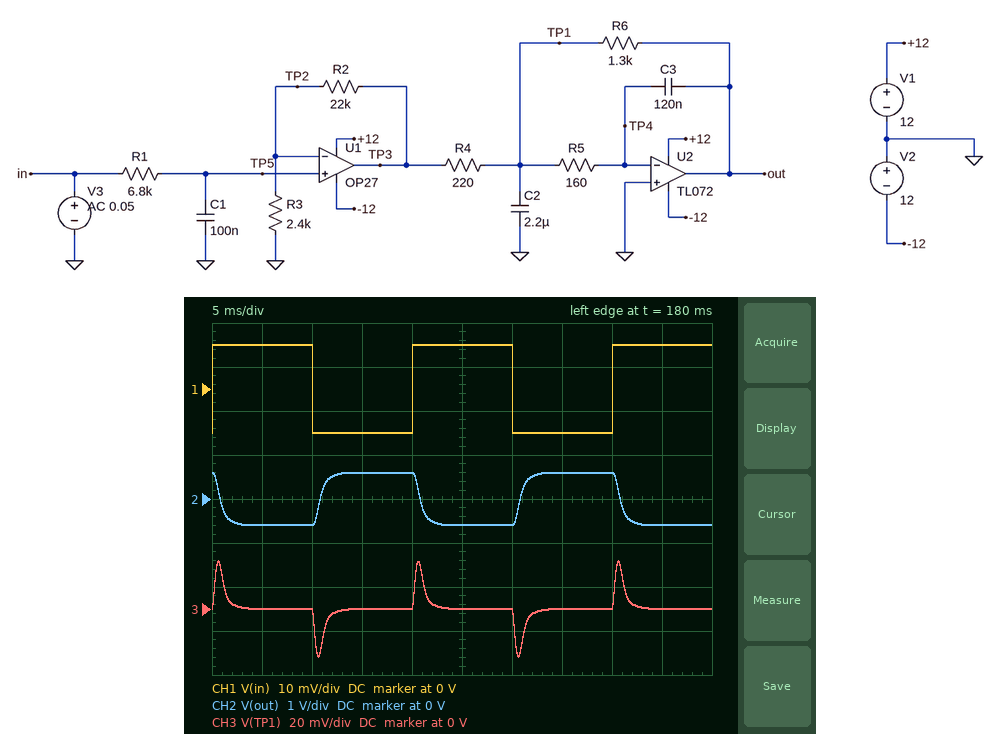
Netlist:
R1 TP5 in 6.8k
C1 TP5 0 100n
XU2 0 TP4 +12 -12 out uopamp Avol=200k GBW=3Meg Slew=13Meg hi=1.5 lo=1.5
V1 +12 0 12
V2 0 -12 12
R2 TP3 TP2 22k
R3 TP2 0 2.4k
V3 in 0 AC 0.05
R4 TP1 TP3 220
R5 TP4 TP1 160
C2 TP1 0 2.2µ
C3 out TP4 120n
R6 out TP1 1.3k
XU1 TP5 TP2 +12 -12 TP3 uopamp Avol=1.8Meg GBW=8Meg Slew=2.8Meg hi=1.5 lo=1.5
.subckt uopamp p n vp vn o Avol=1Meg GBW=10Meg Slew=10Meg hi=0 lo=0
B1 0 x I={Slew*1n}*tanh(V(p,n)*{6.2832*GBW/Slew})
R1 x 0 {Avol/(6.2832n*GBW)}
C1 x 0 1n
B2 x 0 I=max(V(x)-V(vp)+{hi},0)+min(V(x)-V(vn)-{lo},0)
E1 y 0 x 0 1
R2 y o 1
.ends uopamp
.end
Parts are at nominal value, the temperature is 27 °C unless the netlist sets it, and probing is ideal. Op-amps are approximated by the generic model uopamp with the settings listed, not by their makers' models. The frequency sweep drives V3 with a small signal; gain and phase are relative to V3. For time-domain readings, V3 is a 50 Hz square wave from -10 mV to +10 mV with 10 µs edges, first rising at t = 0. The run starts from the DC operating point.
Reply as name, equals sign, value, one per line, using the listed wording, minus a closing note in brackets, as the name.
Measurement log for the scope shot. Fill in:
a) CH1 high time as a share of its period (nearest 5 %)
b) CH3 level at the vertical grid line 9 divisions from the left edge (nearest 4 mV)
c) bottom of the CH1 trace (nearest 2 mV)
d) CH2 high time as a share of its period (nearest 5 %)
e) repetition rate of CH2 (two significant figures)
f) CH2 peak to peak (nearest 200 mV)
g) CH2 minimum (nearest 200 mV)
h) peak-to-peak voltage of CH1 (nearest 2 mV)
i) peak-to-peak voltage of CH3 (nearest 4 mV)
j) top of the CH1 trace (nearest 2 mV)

CH1 high time as a share of its period = 50 %
CH3 level at the vertical grid line 9 divisions from the left edge = 0 V
bottom of the CH1 trace = -10 mV
CH2 high time as a share of its period = 50 %
repetition rate of CH2 = 50 Hz
CH2 peak to peak = 1.2 V
CH2 minimum = -600 mV
peak-to-peak voltage of CH1 = 20 mV
peak-to-peak voltage of CH3 = 44 mV
top of the CH1 trace = 10 mV
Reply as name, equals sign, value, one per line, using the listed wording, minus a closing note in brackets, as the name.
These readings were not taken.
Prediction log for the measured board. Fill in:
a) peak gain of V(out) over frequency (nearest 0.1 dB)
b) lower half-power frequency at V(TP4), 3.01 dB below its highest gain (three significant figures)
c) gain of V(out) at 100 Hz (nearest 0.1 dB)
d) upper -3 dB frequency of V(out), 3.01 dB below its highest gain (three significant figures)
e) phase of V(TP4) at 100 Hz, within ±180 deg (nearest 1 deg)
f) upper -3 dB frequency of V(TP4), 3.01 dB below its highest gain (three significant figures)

peak gain of V(out) over frequency = 35.6 dB
lower half-power frequency at V(TP4), 3.01 dB below its highest gain = 186 Hz
gain of V(out) at 100 Hz = 34.9 dB
upper -3 dB frequency of V(out), 3.01 dB below its highest gain = 245 Hz
phase of V(TP4) at 100 Hz, within ±180 deg = 48 deg
upper -3 dB frequency of V(TP4), 3.01 dB below its highest gain = 804 Hz
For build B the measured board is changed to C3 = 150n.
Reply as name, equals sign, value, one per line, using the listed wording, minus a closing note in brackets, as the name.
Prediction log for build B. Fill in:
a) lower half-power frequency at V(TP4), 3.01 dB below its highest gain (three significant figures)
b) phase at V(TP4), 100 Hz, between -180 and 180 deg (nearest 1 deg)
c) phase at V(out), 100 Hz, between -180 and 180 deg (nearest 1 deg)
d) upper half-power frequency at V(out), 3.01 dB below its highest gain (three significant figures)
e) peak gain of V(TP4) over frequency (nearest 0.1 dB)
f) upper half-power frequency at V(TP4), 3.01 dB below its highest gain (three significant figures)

lower half-power frequency at V(TP4), 3.01 dB below its highest gain = 162 Hz
phase at V(TP4), 100 Hz, between -180 and 180 deg = 45 deg
phase at V(out), 100 Hz, between -180 and 180 deg = 144 deg
upper half-power frequency at V(out), 3.01 dB below its highest gain = 233 Hz
peak gain of V(TP4) over frequency = -48.4 dB
upper half-power frequency at V(TP4), 3.01 dB below its highest gain = 713 Hz
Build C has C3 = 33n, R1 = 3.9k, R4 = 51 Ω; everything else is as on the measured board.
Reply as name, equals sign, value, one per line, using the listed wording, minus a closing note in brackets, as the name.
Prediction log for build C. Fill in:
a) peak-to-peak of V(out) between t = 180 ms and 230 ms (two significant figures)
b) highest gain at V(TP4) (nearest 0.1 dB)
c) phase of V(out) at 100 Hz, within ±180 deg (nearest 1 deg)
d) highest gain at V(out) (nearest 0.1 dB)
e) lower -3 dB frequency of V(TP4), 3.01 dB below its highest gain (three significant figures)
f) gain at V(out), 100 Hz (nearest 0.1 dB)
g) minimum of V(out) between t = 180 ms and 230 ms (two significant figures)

peak-to-peak of V(out) between t = 180 ms and 230 ms = 5.2 V
highest gain at V(TP4) = -30.9 dB
phase of V(out) at 100 Hz, within ±180 deg = 160 deg
highest gain at V(out) = 48.3 dB
lower -3 dB frequency of V(TP4), 3.01 dB below its highest gain = 285 Hz
gain at V(out), 100 Hz = 48.0 dB
minimum of V(out) between t = 180 ms and 230 ms = -2.6 V
